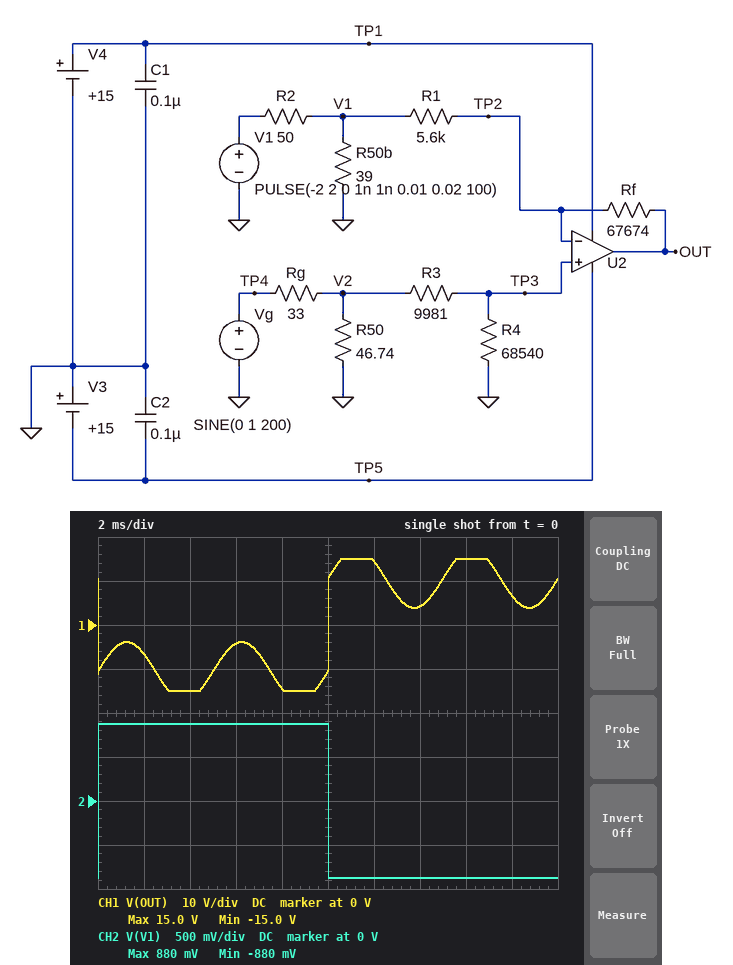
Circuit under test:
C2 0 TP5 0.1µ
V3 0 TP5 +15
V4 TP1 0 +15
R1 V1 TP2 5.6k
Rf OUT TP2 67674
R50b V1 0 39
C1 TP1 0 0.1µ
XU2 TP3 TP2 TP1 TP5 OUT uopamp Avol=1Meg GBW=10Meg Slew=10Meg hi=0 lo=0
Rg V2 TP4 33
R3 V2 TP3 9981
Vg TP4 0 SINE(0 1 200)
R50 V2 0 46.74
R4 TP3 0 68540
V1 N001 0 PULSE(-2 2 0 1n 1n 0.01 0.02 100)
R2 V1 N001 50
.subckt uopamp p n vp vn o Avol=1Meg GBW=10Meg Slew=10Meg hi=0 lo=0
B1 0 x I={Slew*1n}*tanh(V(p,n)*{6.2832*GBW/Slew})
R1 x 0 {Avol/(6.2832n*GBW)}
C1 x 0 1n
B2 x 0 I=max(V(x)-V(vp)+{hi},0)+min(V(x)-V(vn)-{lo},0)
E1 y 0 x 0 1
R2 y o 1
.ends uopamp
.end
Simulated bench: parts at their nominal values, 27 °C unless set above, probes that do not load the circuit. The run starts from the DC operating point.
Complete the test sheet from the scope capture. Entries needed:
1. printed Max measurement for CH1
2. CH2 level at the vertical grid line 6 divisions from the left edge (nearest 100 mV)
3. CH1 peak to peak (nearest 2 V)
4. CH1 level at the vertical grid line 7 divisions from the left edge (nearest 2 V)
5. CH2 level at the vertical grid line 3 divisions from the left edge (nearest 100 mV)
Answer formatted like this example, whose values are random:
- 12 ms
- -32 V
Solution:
- 15.0 V
- -900 mV
- 30 V
- 4 V
- 900 mV
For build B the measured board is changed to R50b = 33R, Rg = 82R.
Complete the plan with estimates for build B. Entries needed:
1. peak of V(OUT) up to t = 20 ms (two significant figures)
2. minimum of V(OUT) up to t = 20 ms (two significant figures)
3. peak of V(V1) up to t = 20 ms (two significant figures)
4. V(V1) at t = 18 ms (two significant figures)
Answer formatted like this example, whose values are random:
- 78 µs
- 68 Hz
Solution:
- 14 V
- -14 V
- 800 mV
- -790 mV
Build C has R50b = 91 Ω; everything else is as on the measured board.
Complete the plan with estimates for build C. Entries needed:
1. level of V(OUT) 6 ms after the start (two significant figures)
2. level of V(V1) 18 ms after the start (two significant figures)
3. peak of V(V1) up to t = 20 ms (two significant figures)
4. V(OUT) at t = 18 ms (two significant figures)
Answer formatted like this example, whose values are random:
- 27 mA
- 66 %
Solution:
- -9.2 V
- -1.3 V
- 1.3 V
- 12 V
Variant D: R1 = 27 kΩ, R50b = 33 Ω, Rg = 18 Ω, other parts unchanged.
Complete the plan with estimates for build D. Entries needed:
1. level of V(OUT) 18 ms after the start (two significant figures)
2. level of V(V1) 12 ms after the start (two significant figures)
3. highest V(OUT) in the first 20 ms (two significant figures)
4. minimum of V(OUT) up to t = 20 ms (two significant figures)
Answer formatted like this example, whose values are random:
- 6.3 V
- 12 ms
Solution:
- 690 mV
- -790 mV
- 4.2 V
- -4.2 V
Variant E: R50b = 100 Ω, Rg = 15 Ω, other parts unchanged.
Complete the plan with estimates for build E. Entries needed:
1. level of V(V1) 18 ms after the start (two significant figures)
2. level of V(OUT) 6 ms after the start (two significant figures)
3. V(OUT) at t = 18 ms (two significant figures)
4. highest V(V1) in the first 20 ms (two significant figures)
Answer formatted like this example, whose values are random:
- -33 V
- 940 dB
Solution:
- -1.3 V
- -7.8 V
- 11 V
- 1.3 V
